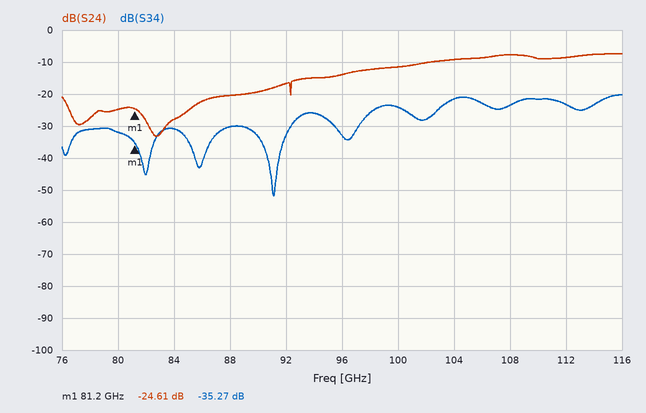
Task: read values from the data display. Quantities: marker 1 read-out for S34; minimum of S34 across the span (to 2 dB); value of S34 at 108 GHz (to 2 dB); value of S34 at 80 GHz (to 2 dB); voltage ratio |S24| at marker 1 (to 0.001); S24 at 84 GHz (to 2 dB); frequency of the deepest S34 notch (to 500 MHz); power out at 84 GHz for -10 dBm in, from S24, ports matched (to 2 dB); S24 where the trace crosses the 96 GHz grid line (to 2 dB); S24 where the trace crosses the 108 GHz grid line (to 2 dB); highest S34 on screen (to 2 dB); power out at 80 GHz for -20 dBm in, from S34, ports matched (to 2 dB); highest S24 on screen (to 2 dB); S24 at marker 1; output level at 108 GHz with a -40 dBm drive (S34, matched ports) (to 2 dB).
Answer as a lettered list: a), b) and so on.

a) -35.27 dB
b) -52 dB
c) -24 dB
d) -32 dB
e) 0.059
f) -28 dB
g) 91.0 GHz
h) -38 dBm
i) -14 dB
j) -8 dB
k) -20 dB
l) -52 dBm
m) -8 dB
n) -24.61 dB
o) -64 dBm
